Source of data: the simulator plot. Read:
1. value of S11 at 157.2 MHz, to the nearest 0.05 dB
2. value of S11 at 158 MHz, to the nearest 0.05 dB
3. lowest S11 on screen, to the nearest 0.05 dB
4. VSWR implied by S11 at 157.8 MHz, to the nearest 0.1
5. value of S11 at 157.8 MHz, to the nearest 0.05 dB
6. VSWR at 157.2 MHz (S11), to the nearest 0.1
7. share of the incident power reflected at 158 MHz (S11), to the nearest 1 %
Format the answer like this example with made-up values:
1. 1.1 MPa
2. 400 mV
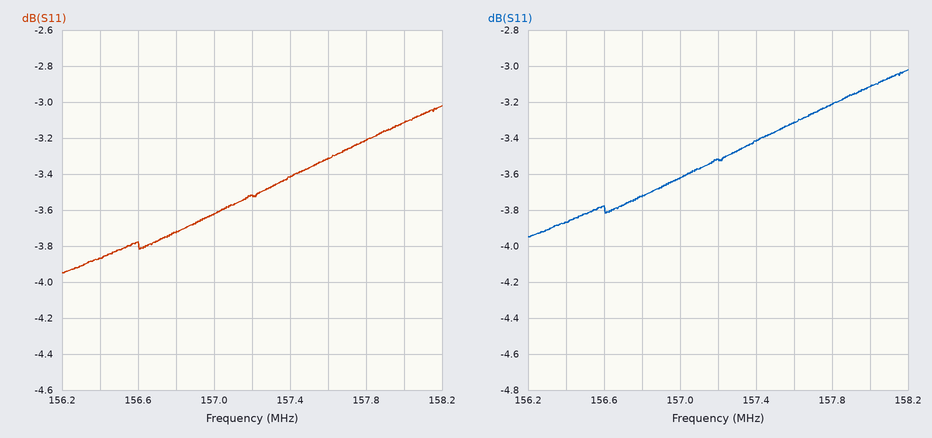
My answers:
1. -3.50 dB
2. -3.10 dB
3. -3.95 dB
4. 5.5
5. -3.20 dB
6. 5.0
7. 49 %
